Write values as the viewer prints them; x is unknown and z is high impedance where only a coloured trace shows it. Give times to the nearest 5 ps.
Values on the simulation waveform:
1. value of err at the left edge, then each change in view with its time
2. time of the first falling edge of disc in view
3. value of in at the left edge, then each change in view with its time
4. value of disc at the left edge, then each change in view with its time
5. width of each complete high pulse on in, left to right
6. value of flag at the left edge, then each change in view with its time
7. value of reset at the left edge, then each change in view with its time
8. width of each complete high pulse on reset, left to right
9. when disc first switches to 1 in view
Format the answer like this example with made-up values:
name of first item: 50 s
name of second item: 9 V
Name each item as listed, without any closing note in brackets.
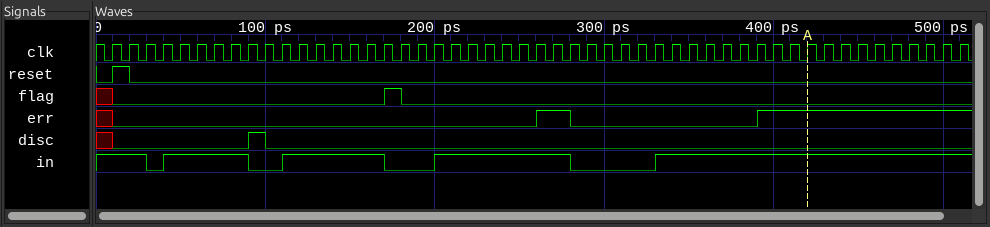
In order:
value of err at the left edge, then each change in view with its time: x, 0 at 10 ps, 1 at 260 ps, 0 at 280 ps, 1 at 390 ps
time of the first falling edge of disc in view: 100 ps
value of in at the left edge, then each change in view with its time: 1, 0 at 30 ps, 1 at 40 ps, 0 at 90 ps, 1 at 110 ps, 0 at 170 ps, 1 at 200 ps, 0 at 280 ps, 1 at 330 ps
value of disc at the left edge, then each change in view with its time: x, 0 at 10 ps, 1 at 90 ps, 0 at 100 ps
width of each complete high pulse on in, left to right: 50 ps, 60 ps, 80 ps
value of flag at the left edge, then each change in view with its time: x, 0 at 10 ps, 1 at 170 ps, 0 at 180 ps
value of reset at the left edge, then each change in view with its time: 0, 1 at 10 ps, 0 at 20 ps
width of each complete high pulse on reset, left to right: 10 ps
when disc first switches to 1 in view: 90 ps
